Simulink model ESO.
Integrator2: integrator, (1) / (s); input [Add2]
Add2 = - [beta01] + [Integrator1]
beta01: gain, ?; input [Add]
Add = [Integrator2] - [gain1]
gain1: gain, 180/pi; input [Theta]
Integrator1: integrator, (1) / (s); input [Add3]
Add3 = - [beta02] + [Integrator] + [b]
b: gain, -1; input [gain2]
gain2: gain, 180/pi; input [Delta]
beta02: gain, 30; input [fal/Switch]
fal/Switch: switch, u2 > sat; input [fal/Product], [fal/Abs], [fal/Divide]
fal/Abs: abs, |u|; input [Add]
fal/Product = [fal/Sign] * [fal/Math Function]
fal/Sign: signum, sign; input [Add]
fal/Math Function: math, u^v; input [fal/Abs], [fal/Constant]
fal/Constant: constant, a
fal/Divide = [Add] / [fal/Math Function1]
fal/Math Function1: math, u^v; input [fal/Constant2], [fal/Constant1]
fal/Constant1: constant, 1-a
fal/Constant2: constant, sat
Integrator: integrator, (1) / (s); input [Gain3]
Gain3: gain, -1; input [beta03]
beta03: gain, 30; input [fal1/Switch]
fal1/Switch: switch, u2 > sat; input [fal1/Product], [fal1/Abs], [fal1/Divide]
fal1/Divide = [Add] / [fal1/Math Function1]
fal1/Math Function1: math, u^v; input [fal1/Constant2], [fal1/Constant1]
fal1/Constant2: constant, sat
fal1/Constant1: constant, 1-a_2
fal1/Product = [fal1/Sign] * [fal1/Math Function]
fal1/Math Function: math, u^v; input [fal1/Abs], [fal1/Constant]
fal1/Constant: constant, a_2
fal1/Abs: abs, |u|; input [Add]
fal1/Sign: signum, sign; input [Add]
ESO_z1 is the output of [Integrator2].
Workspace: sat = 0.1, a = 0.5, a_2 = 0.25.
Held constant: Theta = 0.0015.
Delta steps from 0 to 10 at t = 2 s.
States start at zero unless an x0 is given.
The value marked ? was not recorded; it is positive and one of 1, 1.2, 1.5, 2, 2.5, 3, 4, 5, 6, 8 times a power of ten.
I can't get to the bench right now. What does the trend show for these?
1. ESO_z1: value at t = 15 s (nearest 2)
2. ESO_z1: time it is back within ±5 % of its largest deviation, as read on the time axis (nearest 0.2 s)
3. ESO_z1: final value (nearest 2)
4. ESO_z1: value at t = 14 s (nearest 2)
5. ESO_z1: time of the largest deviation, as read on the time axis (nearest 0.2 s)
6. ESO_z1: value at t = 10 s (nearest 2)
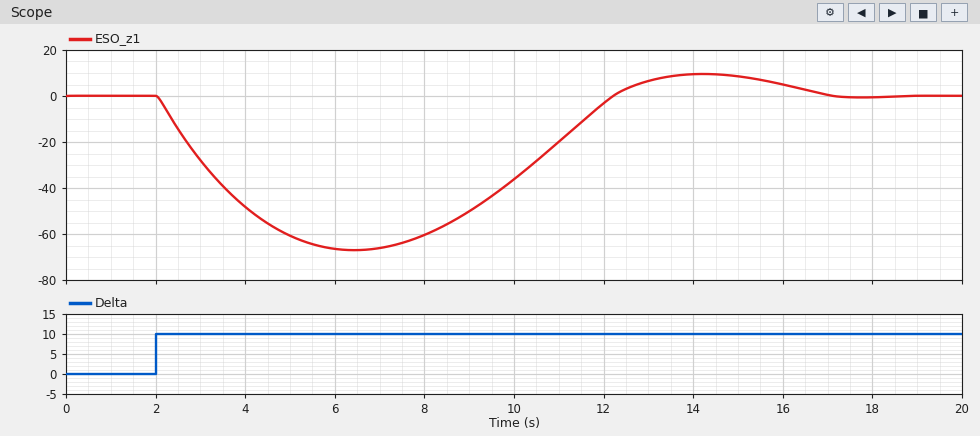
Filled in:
8
16.4 s
0
10
6.4 s
-36
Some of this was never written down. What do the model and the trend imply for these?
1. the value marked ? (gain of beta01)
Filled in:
15
